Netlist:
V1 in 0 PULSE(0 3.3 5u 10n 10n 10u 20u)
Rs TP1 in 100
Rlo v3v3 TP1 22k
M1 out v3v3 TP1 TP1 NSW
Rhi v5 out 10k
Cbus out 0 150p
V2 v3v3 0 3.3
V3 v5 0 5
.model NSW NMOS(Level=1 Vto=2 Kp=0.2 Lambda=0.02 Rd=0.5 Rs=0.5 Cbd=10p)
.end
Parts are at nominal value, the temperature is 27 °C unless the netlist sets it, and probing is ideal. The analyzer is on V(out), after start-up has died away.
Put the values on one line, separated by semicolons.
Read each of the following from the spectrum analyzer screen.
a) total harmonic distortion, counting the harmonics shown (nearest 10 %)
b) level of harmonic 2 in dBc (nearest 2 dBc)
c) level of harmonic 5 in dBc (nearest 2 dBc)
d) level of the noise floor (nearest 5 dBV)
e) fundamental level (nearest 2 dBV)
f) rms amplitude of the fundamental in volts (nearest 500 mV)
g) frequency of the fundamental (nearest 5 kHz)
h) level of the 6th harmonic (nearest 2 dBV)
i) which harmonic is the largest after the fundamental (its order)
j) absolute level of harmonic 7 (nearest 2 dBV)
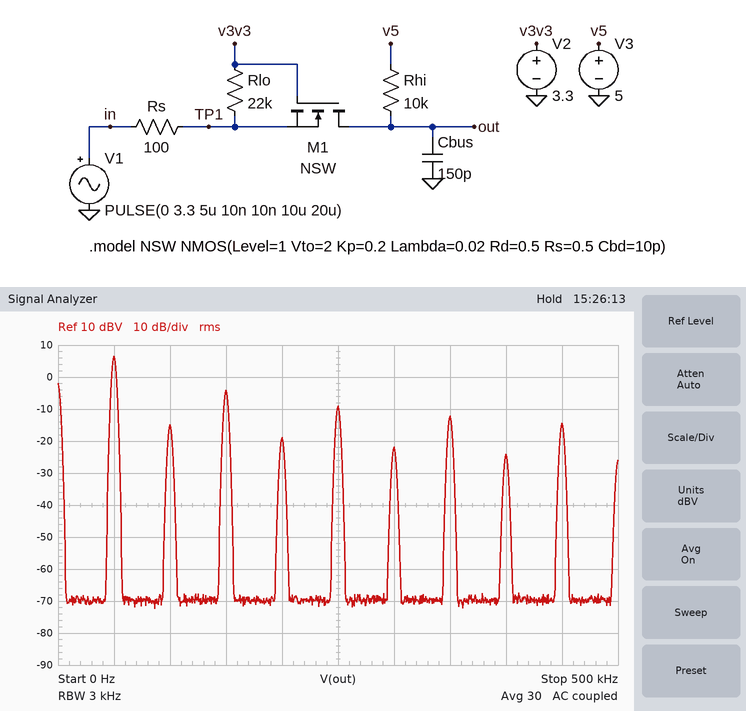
40 %; -22 dBc; -16 dBc; -70 dBV; 6 dBV; 2.0 V; 50 kHz; -22 dBV; 3; -12 dBV
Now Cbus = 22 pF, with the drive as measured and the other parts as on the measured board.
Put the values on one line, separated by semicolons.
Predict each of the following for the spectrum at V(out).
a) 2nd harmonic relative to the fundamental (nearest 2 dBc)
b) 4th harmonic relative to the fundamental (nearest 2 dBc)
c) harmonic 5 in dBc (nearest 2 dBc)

-34 dBc; -34 dBc; -14 dBc
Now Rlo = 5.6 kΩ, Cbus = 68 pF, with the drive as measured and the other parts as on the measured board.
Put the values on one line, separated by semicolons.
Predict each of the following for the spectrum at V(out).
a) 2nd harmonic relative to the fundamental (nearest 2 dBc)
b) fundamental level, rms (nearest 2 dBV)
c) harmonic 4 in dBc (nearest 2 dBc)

-26 dBc; 6 dBV; -28 dBc
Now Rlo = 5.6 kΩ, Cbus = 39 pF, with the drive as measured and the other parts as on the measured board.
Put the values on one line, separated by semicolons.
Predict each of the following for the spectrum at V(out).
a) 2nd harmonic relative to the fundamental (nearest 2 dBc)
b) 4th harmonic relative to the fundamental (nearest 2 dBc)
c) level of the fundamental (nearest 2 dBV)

-30 dBc; -30 dBc; 6 dBV
